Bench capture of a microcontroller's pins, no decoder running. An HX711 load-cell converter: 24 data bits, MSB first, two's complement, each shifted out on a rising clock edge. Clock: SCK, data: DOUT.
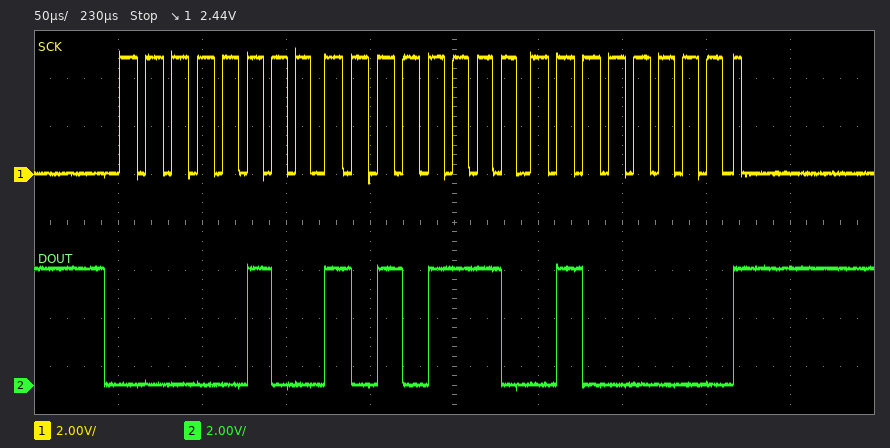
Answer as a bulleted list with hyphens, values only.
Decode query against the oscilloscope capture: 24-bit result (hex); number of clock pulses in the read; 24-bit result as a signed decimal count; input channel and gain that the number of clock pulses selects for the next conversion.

- 0x04AE40
- 25
- 306752
- channel A, gain 128
